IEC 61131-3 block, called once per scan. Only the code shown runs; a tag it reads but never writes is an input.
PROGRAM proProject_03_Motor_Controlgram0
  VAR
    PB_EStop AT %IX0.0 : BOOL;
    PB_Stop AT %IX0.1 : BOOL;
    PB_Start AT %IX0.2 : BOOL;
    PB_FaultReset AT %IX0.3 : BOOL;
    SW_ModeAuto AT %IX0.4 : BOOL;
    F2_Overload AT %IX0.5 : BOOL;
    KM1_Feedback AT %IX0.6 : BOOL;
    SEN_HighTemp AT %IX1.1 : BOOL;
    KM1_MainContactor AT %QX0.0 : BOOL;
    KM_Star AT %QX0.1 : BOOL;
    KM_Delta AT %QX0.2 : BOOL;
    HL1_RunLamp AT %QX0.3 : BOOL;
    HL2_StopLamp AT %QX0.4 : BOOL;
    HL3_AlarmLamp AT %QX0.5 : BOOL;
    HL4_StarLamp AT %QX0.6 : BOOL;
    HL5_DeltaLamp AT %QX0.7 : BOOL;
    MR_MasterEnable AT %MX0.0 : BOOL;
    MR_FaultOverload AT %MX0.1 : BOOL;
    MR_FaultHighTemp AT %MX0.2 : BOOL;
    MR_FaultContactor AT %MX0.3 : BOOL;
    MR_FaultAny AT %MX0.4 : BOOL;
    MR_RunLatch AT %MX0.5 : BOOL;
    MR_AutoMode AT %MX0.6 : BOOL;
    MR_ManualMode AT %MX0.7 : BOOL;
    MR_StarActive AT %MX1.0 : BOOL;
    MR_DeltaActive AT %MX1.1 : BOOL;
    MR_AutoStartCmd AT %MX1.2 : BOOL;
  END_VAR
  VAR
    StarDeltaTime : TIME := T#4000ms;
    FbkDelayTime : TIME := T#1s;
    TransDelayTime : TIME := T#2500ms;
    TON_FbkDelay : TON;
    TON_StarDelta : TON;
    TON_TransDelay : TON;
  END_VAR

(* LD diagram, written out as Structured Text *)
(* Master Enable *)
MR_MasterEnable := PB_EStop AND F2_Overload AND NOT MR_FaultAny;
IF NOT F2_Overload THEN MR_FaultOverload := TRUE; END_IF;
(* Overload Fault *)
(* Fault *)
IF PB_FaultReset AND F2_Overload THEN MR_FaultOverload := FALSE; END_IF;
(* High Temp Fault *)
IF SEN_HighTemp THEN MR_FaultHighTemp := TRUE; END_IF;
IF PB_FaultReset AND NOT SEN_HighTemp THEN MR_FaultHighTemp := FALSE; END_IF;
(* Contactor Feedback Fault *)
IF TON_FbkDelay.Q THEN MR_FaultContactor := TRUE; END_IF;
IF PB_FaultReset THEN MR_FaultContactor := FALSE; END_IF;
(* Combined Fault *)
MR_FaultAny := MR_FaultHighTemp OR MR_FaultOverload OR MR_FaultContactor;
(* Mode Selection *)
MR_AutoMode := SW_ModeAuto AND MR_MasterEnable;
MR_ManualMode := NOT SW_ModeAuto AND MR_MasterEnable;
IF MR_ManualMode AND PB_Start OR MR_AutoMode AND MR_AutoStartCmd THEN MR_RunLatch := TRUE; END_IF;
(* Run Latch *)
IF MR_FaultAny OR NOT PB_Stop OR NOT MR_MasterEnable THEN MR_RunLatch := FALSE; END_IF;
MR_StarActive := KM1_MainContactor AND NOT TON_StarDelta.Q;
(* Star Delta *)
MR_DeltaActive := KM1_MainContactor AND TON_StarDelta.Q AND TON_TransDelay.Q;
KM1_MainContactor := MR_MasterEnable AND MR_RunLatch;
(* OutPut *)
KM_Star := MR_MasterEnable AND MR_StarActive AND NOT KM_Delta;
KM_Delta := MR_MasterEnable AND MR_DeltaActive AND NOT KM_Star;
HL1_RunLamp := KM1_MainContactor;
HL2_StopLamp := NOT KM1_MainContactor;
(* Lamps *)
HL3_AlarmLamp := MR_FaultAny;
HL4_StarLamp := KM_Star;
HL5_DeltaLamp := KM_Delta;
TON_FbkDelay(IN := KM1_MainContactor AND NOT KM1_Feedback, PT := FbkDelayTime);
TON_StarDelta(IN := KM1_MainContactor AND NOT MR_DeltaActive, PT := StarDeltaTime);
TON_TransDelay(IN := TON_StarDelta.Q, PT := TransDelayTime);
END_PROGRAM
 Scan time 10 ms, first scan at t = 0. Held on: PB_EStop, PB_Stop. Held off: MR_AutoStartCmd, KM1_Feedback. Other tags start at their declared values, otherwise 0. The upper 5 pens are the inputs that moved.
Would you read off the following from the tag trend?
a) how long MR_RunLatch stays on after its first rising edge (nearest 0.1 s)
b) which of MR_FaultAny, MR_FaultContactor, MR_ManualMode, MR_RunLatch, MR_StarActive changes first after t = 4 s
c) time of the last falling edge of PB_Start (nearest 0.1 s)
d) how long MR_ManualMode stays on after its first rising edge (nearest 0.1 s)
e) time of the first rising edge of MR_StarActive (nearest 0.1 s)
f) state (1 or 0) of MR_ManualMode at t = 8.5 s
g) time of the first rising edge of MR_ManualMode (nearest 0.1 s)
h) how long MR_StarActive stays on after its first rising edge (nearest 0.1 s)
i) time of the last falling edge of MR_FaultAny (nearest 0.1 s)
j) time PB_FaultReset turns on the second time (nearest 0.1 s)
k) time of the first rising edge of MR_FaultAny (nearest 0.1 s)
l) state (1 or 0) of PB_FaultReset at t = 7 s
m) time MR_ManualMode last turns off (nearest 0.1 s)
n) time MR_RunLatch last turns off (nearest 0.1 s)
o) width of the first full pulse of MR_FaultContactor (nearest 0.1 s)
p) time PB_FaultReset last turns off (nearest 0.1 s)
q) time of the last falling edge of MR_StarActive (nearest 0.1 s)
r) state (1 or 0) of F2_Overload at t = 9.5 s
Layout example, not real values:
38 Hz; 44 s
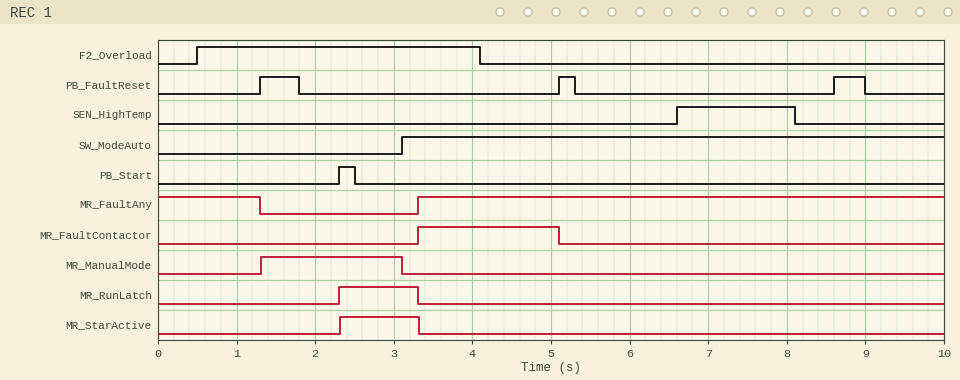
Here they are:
1.0 s; MR_FaultContactor; 2.5 s; 1.8 s; 2.3 s; 0; 1.3 s; 1.0 s; 1.3 s; 5.1 s; 3.3 s; 0; 3.1 s; 3.3 s; 1.8 s; 9.0 s; 3.3 s; 0
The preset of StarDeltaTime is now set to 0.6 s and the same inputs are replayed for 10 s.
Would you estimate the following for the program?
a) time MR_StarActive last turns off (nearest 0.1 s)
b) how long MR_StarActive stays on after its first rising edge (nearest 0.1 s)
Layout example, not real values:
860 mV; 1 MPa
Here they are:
2.9 s; 0.6 s
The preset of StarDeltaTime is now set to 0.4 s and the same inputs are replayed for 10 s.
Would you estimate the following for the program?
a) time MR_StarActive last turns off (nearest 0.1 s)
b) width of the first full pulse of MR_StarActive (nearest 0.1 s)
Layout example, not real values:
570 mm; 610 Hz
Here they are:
2.7 s; 0.4 s
